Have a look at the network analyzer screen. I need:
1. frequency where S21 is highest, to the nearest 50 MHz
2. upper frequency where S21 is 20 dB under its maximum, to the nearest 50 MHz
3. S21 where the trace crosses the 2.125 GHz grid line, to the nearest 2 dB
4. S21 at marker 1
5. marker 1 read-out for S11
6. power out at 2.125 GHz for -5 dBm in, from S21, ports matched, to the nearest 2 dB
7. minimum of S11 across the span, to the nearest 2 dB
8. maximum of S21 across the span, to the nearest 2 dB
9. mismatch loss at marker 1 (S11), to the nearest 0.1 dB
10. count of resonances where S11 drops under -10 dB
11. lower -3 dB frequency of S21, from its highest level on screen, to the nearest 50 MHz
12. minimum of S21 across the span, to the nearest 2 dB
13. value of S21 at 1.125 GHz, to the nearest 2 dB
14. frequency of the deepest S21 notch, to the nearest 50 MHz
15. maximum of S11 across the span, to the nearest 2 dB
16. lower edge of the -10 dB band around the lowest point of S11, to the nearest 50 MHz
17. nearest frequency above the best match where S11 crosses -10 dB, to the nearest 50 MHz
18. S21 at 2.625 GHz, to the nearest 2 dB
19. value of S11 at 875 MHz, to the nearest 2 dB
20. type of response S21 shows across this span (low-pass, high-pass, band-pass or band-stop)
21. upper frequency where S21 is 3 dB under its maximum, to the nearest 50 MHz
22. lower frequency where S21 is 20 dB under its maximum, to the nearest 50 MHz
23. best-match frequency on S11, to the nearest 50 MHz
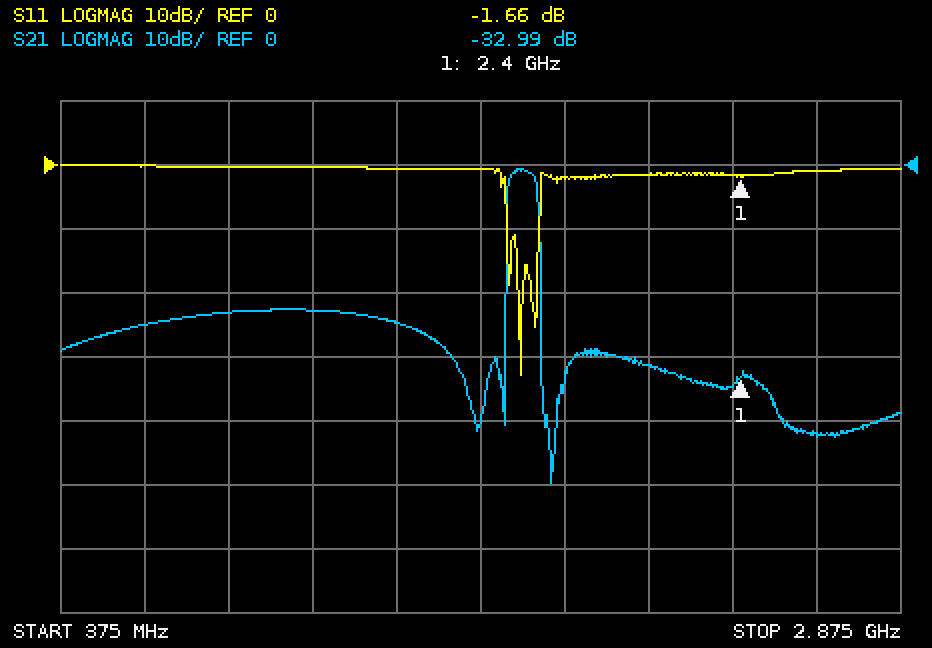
1.75 GHz
1.80 GHz
-32 dB
-32.99 dB
-1.66 dB
-36 dBm
-32 dB
0 dB
5.0 dB
3
1.70 GHz
-50 dB
-22 dB
1.85 GHz
0 dB
1.70 GHz
1.80 GHz
-42 dB
0 dB
band-pass
1.80 GHz
1.70 GHz
1.75 GHz
